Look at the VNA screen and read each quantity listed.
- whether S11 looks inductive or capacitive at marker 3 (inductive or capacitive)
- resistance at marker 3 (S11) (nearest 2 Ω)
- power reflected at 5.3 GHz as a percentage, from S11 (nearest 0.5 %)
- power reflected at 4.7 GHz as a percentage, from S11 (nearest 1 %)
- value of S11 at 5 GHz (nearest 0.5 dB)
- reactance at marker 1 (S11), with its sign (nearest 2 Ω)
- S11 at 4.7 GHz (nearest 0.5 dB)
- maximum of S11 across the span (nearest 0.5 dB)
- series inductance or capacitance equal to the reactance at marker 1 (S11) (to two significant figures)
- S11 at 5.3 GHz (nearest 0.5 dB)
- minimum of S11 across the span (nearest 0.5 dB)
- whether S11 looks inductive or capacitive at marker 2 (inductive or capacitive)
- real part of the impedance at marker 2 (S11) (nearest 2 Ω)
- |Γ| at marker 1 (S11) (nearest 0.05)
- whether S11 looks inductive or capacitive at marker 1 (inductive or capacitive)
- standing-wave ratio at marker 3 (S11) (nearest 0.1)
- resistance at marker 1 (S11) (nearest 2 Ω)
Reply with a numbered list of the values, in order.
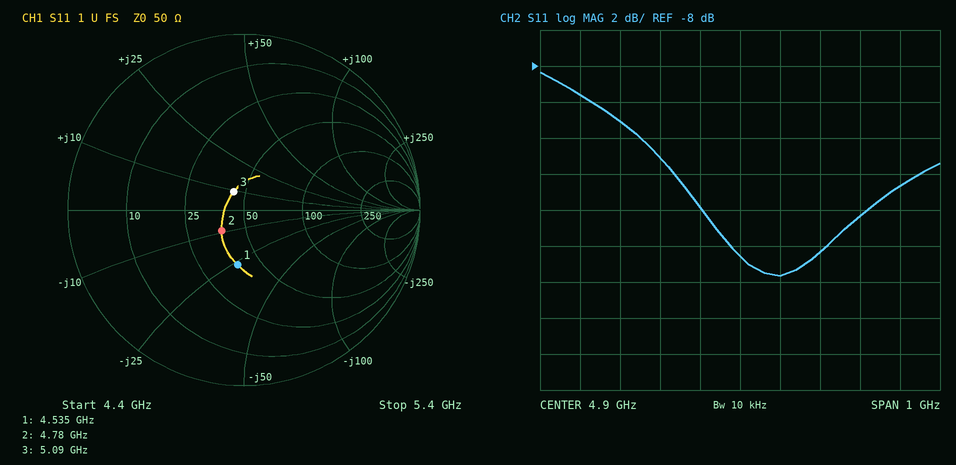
1. inductive
2. 44 Ω
3. 3.5 %
4. 5 %
5. -19.5 dB
6. -26 Ω
7. -13.0 dB
8. -8.5 dB
9. 1.3 pF
10. -14.5 dB
11. -19.5 dB
12. capacitive
13. 38 Ω
14. 0.30
15. capacitive
16. 1.3
17. 38 Ω
